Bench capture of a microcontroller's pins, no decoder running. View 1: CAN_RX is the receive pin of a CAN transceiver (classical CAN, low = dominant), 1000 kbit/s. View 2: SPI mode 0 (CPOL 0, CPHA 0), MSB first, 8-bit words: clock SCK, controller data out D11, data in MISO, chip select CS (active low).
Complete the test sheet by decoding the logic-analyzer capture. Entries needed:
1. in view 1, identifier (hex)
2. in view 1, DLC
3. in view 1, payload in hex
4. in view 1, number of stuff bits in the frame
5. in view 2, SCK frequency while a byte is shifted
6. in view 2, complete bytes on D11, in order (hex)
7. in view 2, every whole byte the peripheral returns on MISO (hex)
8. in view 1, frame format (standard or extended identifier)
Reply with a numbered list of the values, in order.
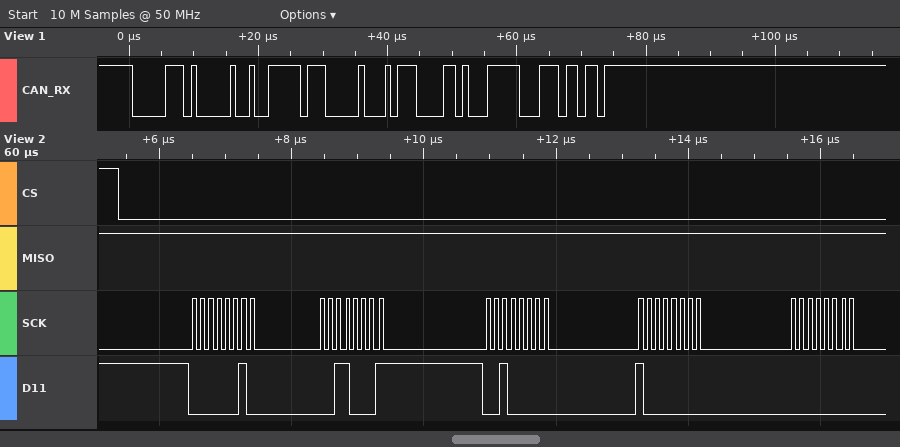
1. 0x068
2. 4
3. FF 00 B8 68
4. 5
5. 8 MHz
6. 02 31 20 80 00
7. FF FF FF FF FF
8. standard
